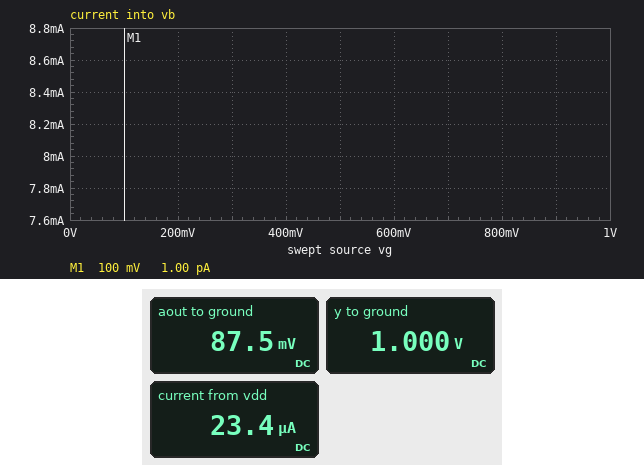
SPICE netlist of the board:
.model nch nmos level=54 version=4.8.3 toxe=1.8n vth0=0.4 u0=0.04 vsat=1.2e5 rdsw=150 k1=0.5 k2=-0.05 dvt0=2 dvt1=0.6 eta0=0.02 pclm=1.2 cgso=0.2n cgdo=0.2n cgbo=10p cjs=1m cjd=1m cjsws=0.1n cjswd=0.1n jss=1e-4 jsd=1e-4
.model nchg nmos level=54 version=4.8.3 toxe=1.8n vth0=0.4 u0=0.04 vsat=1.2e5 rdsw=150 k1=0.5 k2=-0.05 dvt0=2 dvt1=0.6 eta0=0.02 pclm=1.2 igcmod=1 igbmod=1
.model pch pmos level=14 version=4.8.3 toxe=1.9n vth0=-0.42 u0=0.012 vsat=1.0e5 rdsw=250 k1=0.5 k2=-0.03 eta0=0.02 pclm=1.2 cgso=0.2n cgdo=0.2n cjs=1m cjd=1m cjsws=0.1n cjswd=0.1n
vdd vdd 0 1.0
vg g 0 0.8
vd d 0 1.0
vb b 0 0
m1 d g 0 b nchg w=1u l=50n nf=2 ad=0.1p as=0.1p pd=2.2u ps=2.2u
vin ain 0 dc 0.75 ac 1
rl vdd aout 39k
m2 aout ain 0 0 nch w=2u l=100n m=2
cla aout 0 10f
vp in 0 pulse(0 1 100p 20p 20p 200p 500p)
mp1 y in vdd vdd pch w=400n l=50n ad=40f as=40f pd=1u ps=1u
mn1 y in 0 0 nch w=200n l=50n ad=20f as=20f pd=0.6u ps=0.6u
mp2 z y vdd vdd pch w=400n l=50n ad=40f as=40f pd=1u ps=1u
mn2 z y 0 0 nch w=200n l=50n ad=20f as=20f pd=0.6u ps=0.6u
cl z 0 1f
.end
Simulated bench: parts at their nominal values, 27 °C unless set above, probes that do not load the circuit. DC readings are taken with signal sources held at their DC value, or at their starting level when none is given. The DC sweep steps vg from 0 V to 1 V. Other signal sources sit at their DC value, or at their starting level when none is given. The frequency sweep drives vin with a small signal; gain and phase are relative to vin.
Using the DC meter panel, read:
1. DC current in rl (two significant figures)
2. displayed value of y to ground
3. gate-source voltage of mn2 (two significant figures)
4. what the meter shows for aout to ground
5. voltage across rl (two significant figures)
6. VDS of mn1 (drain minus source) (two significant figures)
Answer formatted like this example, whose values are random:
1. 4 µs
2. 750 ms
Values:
1. 23 µA
2. 1.000 V
3. 1.0 V
4. 87.5 mV
5. 910 mV
6. 1.0 V
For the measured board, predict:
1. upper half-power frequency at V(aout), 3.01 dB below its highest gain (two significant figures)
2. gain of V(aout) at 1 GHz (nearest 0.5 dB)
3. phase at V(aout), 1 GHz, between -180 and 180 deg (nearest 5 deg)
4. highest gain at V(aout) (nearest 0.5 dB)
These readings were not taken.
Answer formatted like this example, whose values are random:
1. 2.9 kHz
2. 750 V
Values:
1. 1.5 GHz
2. 12.0 dB
3. 145 deg
4. 13.5 dB
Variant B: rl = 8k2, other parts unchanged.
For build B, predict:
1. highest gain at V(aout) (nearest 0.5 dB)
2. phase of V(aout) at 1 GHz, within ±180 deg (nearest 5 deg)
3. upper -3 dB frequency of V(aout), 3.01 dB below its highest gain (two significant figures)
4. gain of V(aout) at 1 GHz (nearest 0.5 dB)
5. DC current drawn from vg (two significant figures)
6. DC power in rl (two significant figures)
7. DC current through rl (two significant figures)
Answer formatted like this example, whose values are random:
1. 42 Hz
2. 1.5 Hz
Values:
1. 16.0 dB
2. 155 deg
3. 2.2 GHz
4. 15.0 dB
5. 320 mA
6. 18 µW
7. 47 µA
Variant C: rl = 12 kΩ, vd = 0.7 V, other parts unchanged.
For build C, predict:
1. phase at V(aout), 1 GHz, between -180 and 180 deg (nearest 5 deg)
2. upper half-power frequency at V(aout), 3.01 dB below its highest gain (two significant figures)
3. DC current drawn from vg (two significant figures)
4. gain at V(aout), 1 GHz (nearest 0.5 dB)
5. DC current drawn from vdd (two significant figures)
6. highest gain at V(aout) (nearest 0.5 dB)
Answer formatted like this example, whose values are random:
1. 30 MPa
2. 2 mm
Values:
1. 150 deg
2. 1.7 GHz
3. 260 mA
4. 16.0 dB
5. 42 µA
6. 17.5 dB
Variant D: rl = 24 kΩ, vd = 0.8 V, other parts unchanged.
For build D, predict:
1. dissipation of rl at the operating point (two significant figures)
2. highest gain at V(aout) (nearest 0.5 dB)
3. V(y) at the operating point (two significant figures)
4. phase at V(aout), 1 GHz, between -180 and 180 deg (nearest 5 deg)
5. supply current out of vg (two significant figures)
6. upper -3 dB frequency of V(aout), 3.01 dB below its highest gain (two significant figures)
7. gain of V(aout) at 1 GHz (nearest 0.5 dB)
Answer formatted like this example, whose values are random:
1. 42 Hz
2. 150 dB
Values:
1. 24 µW
2. 18.5 dB
3. 1.0 V
4. 135 deg
5. 280 mA
6. 1.1 GHz
7. 16.0 dB
